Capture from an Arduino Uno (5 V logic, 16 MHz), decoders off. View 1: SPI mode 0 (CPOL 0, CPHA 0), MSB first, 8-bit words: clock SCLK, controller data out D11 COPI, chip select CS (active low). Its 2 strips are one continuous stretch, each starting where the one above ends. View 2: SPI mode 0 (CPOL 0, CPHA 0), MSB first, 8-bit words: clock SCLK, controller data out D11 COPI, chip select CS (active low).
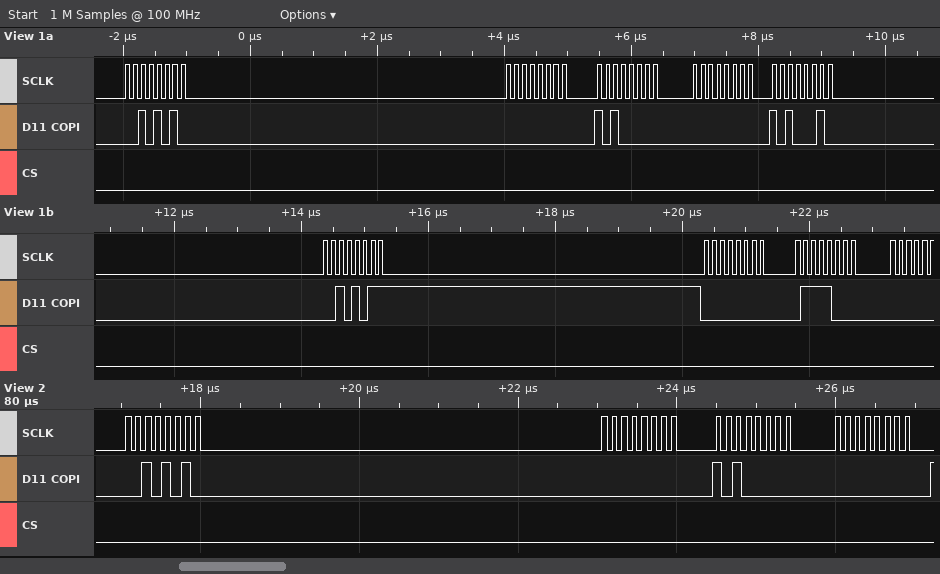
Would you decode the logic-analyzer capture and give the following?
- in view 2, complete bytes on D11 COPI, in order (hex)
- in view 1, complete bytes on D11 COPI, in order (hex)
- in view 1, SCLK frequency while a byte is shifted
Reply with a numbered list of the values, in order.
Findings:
1. 2A 00 A0 00
2. 2A 00 A0 00 A2 2B 00 78
3. 8 MHz
